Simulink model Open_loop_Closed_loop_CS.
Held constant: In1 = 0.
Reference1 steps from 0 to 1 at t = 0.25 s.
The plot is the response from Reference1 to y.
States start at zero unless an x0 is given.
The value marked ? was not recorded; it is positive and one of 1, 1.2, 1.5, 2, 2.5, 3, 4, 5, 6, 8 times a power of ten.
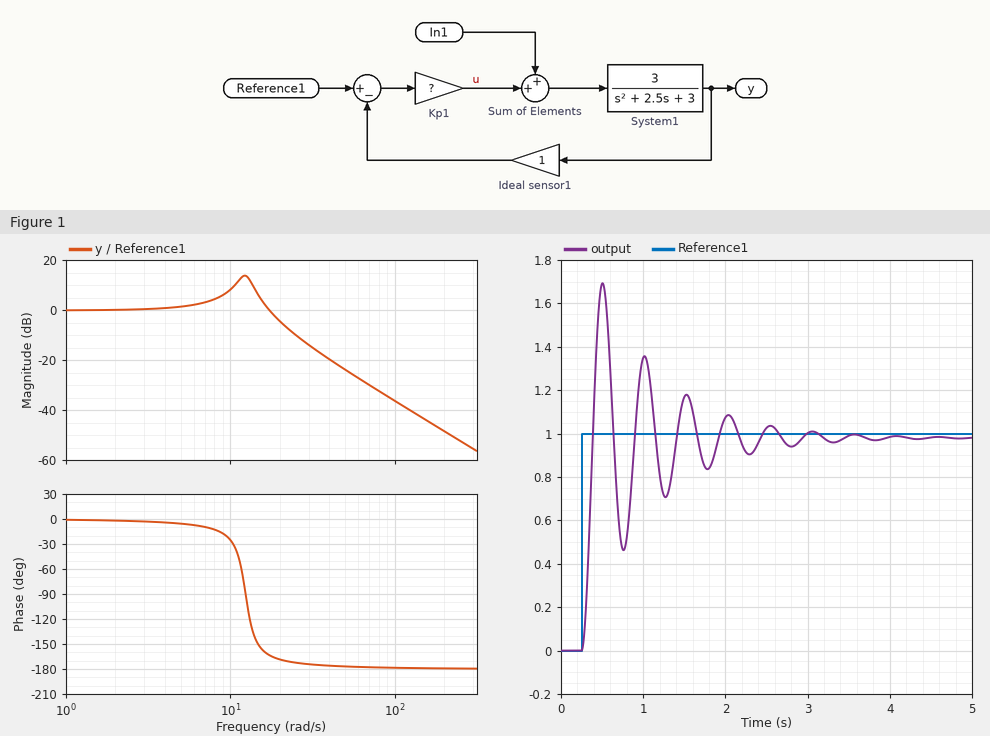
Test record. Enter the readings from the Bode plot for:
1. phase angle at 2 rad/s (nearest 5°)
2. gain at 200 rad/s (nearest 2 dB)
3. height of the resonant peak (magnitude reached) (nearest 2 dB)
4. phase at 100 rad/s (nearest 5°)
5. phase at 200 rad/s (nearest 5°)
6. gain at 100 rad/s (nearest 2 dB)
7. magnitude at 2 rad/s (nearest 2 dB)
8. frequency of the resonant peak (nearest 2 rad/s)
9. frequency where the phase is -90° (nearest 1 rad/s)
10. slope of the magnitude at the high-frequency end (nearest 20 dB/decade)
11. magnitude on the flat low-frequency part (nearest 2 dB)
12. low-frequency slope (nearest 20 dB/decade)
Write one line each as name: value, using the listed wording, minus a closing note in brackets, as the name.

phase angle at 2 rad/s: 0°
gain at 200 rad/s: -48 dB
height of the resonant peak (magnitude reached): 14 dB
phase at 100 rad/s: -180°
phase at 200 rad/s: -180°
gain at 100 rad/s: -36 dB
magnitude at 2 rad/s: 0 dB
frequency of the resonant peak: 12 rad/s
frequency where the phase is -90°: 12 rad/s
slope of the magnitude at the high-frequency end: -40 dB/decade
magnitude on the flat low-frequency part: 0 dB
low-frequency slope: 0 dB/decade
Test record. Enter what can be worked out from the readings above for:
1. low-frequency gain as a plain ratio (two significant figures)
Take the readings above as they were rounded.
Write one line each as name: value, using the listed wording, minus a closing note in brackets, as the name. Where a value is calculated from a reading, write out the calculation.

low-frequency gain as a plain ratio: 10^(0 / 20) = 1.0
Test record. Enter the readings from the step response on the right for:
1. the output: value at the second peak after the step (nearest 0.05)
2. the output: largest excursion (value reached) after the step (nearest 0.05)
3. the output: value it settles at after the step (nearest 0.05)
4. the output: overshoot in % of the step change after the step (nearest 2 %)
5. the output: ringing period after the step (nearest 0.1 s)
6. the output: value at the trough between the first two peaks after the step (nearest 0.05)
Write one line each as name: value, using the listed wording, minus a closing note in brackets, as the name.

the output: value at the second peak after the step: 1.35
the output: largest excursion (value reached) after the step: 1.70
the output: value it settles at after the step: 1.00
the output: overshoot in % of the step change after the step: 72 %
the output: ringing period after the step: 0.5 s
the output: value at the trough between the first two peaks after the step: 0.45
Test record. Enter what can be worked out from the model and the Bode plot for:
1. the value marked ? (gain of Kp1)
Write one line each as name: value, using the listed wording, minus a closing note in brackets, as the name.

the value marked ?: 50
